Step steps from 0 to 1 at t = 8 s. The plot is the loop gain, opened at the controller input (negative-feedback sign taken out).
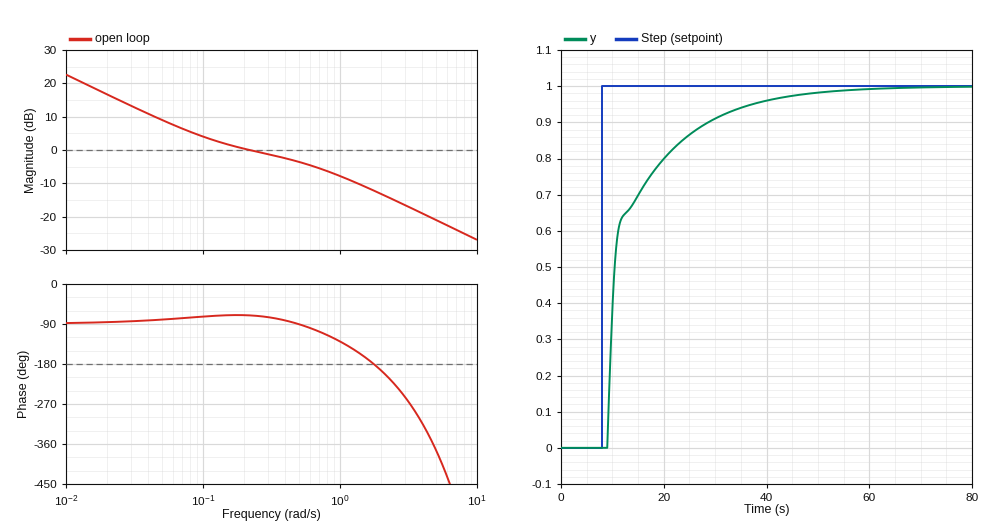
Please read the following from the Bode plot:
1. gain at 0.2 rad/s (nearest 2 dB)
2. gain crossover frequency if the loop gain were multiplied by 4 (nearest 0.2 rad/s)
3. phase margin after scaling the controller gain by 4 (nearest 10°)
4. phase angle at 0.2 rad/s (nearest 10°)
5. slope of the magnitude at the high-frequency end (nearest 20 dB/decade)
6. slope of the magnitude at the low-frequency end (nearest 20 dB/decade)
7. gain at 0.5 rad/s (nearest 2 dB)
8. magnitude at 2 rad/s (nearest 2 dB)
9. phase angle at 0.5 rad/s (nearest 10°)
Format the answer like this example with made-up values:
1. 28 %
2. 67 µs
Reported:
1. 0 dB
2. 1.8 rad/s
3. 0°
4. -70°
5. -20 dB/decade
6. -20 dB/decade
7. -4 dB
8. -14 dB
9. -90°
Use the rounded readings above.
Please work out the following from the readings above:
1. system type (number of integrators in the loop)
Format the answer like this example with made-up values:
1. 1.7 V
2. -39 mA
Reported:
1. 1
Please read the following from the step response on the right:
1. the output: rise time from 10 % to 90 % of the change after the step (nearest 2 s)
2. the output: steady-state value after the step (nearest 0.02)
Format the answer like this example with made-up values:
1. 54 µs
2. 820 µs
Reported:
1. 20 s
2. 1.00
